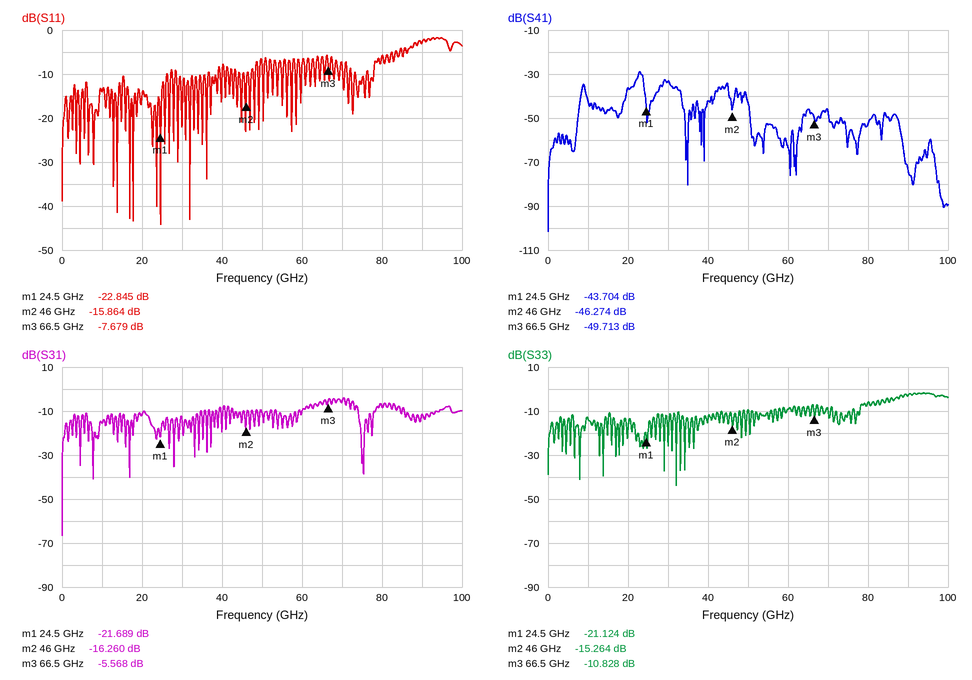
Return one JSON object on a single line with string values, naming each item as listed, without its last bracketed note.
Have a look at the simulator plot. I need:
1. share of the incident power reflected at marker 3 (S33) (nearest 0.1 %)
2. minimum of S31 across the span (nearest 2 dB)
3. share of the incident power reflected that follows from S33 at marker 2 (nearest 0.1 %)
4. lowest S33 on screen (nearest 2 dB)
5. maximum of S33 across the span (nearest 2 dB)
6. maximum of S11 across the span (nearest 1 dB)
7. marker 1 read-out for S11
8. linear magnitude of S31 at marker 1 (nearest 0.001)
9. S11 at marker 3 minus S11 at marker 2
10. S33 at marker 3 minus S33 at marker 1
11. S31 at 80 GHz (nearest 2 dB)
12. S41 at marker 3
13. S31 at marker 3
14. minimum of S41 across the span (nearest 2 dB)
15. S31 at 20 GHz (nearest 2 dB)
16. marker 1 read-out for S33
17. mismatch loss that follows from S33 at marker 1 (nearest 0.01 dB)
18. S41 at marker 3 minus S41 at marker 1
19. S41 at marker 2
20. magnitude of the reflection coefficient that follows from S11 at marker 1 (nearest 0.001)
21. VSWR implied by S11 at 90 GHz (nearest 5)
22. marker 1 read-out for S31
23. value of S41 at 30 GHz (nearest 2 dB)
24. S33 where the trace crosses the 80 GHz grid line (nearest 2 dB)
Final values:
{"share of the incident power reflected at marker 3 (S33)": "8.3 %", "minimum of S31 across the span": "-66 dB", "share of the incident power reflected that follows from S33 at marker 2": "3.0 %", "lowest S33 on screen": "-44 dB", "maximum of S33 across the span": "-2 dB", "maximum of S11 across the span": "-2 dB", "marker 1 read-out for S11": "-22.845 dB", "linear magnitude of S31 at marker 1": "0.082", "S11 at marker 3 minus S11 at marker 2": "8.185 dB", "S33 at marker 3 minus S33 at marker 1": "10.296 dB", "S31 at 80 GHz": "-8 dB", "S41 at marker 3": "-49.713 dB", "S31 at marker 3": "-5.568 dB", "minimum of S41 across the span": "-102 dB", "S31 at 20 GHz": "-12 dB", "marker 1 read-out for S33": "-21.124 dB", "mismatch loss that follows from S33 at marker 1": "0.03 dB", "S41 at marker 3 minus S41 at marker 1": "-6.009 dB", "S41 at marker 2": "-46.274 dB", "magnitude of the reflection coefficient that follows from S11 at marker 1": "0.072", "VSWR implied by S11 at 90 GHz": "5", "marker 1 read-out for S31": "-21.689 dB", "value of S41 at 30 GHz": "-34 dB", "S33 where the trace crosses the 80 GHz grid line": "-6 dB"}
